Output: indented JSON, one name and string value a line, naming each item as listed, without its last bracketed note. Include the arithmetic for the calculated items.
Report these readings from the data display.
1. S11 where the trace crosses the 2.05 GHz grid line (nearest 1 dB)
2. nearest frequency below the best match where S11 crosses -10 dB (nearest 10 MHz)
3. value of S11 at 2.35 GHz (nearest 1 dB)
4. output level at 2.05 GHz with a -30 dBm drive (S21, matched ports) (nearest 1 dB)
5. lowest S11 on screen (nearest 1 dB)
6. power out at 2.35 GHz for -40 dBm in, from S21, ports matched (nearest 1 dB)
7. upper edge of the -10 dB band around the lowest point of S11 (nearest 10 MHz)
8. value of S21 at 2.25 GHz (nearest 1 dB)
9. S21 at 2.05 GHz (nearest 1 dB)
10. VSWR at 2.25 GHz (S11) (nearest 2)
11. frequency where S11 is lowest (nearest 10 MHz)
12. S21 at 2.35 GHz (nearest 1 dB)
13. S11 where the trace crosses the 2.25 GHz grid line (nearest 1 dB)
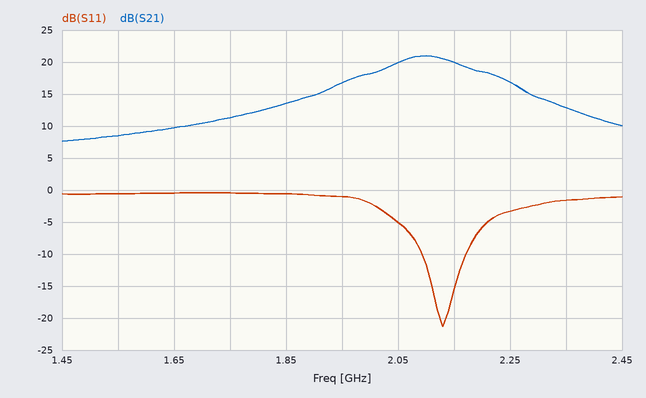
{
  "S11 where the trace crosses the 2.05 GHz grid line": "-5 dB",
  "nearest frequency below the best match where S11 crosses -10 dB": "2.09 GHz",
  "value of S11 at 2.35 GHz": "-2 dB",
  "output level at 2.05 GHz with a -30 dBm drive (S21, matched ports)": "-30 dBm + (20 dB) = -10 dBm",
  "lowest S11 on screen": "-21 dB",
  "power out at 2.35 GHz for -40 dBm in, from S21, ports matched": "-40 dBm + (13 dB) = -27 dBm",
  "upper edge of the -10 dB band around the lowest point of S11": "2.17 GHz",
  "value of S21 at 2.25 GHz": "17 dB",
  "S21 at 2.05 GHz": "20 dB",
  "VSWR at 2.25 GHz (S11)": "|Γ| = 10^(-3/20) = 0.7079; VSWR = (1 + 0.7079)/(1 − 0.7079) ≈ 6",
  "frequency where S11 is lowest": "2.13 GHz",
  "S21 at 2.35 GHz": "13 dB",
  "S11 where the trace crosses the 2.25 GHz grid line": "-3 dB"
}
